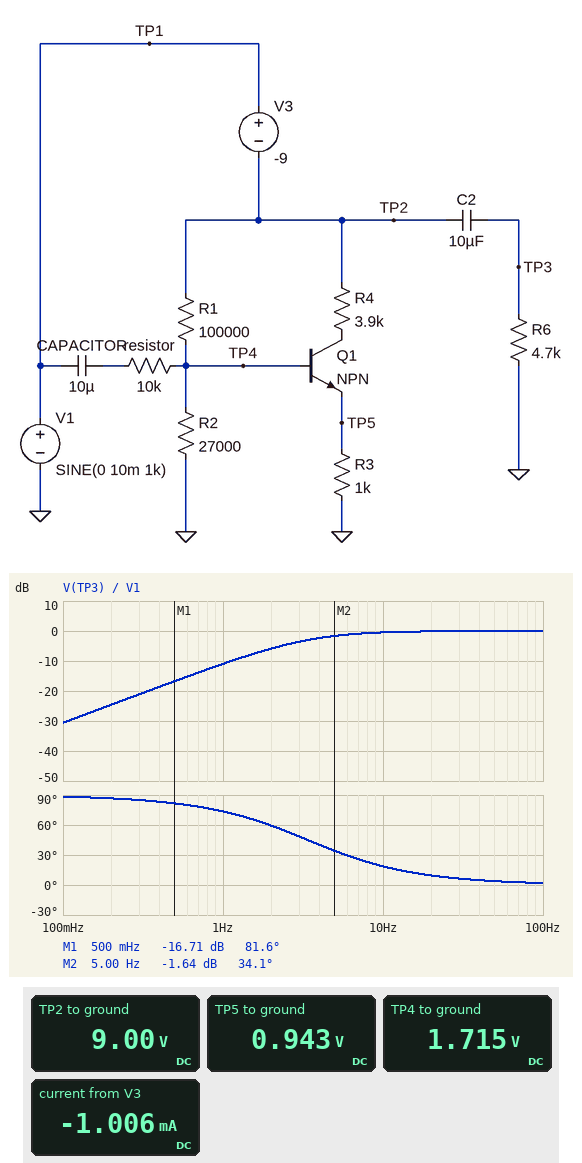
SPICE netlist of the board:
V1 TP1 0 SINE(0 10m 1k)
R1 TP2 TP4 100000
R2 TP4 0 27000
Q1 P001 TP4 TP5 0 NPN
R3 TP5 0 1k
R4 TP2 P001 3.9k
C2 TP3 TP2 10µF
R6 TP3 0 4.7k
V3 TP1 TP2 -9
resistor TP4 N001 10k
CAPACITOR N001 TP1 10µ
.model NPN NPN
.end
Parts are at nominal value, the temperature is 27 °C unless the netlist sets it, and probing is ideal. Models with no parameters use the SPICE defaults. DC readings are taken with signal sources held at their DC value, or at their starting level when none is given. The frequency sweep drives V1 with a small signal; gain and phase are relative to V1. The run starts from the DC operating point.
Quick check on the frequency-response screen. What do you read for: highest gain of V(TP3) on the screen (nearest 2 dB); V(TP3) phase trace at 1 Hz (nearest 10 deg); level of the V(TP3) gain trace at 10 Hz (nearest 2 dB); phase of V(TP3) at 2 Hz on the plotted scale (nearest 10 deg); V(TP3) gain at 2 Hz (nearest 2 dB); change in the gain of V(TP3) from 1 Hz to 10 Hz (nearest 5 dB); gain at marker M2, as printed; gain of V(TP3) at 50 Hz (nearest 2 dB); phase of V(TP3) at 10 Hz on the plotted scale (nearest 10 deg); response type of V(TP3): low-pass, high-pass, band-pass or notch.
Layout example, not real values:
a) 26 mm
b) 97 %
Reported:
a) 0 dB
b) 70 deg
c) 0 dB
d) 60 deg
e) -6 dB
f) 10 dB
g) -1.64 dB
h) 0 dB
i) 20 deg
j) high-pass
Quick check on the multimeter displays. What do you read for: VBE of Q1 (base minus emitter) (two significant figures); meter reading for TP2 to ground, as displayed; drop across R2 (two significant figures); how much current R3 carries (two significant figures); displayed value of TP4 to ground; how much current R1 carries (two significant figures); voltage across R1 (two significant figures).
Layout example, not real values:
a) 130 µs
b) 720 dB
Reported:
a) 770 mV
b) 9.00 V
c) 1.7 V
d) 940 µA
e) 1.715 V
f) 73 µA
g) 7.3 V
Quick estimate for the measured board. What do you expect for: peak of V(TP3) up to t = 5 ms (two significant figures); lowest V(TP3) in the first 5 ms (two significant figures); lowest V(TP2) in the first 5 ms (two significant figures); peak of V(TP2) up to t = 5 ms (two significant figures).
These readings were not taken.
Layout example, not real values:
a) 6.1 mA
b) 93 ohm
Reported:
a) 10 mV
b) -10 mV
c) 9.0 V
d) 9.0 V
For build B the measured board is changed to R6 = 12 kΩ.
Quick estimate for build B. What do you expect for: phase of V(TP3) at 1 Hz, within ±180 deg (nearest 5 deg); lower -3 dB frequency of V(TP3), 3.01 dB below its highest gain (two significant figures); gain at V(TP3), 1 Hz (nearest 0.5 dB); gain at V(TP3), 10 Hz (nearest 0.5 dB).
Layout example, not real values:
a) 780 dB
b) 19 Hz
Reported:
a) 55 deg
b) 1.3 Hz
c) -4.5 dB
d) 0 dB
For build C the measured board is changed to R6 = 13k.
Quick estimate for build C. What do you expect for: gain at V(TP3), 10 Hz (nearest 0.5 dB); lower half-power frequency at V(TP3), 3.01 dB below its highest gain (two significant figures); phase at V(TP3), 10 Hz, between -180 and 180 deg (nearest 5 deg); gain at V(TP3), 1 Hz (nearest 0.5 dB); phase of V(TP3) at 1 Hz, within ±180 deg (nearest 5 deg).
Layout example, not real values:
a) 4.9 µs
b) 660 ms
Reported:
a) 0 dB
b) 1.2 Hz
c) 5 deg
d) -4.0 dB
e) 50 deg
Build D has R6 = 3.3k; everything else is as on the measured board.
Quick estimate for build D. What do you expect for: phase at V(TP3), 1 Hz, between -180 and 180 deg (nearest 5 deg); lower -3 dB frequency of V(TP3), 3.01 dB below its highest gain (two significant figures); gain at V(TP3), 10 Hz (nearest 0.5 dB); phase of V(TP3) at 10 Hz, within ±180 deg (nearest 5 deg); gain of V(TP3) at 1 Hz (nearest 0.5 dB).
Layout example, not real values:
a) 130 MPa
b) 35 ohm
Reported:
a) 80 deg
b) 4.8 Hz
c) -1.0 dB
d) 25 deg
e) -14.0 dB
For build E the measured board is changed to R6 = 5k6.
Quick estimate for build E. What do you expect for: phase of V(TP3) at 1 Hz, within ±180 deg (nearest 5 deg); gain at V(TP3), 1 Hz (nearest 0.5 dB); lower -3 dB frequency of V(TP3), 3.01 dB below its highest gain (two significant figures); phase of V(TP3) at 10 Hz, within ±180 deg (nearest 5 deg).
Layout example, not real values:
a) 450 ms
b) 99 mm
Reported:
a) 70 deg
b) -9.5 dB
c) 2.8 Hz
d) 15 deg
